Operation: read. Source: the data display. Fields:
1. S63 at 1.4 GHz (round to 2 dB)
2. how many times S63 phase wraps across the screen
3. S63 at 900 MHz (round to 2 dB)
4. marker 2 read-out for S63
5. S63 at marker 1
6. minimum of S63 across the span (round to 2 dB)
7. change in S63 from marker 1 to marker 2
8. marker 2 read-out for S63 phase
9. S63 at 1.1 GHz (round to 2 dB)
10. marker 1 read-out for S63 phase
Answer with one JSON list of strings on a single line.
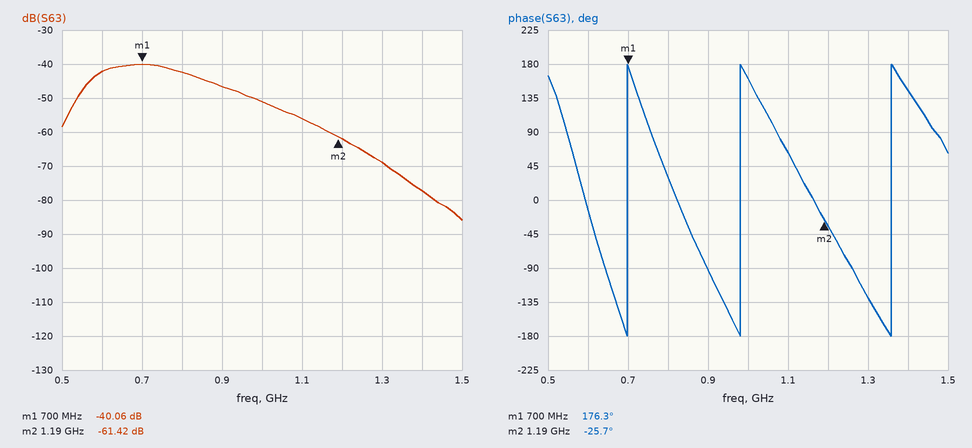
["-78 dB", "3", "-46 dB", "-61.42 dB", "-40.06 dB", "-86 dB", "-21.36 dB", "-25.7°", "-56 dB", "176.3°"]
